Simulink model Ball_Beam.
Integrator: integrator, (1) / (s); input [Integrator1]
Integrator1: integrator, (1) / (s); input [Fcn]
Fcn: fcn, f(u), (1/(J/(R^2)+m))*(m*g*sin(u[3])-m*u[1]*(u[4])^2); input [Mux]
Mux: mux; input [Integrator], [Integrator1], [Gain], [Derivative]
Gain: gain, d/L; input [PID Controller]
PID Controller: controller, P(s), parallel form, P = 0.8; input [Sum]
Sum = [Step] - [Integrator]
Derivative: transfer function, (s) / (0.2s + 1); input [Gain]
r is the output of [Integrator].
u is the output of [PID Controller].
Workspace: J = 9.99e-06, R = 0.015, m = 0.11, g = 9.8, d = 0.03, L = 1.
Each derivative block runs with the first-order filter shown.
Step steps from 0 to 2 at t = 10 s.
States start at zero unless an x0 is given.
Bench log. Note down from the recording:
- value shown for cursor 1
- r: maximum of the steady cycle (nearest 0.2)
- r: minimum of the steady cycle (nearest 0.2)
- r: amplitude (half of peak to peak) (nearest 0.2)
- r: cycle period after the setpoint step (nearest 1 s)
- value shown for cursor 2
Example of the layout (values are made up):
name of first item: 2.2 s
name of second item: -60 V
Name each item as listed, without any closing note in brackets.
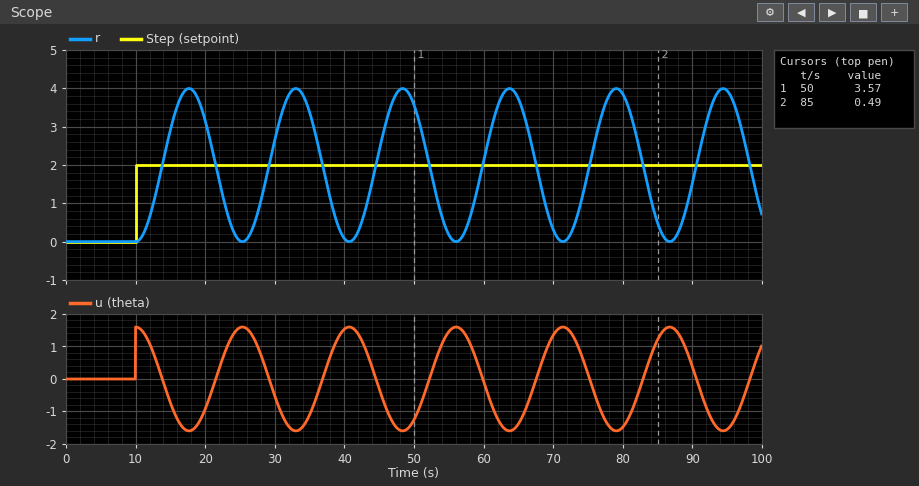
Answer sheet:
value shown for cursor 1: 3.57
r: maximum of the steady cycle: 4.0
r: minimum of the steady cycle: 0.0
r: amplitude (half of peak to peak): 2.0
r: cycle period after the setpoint step: 15 s
value shown for cursor 2: 0.49
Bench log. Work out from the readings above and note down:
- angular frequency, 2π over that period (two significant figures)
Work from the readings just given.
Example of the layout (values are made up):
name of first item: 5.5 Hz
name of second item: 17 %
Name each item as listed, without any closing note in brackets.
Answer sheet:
angular frequency, 2π over that period: 0.42 rad/s
